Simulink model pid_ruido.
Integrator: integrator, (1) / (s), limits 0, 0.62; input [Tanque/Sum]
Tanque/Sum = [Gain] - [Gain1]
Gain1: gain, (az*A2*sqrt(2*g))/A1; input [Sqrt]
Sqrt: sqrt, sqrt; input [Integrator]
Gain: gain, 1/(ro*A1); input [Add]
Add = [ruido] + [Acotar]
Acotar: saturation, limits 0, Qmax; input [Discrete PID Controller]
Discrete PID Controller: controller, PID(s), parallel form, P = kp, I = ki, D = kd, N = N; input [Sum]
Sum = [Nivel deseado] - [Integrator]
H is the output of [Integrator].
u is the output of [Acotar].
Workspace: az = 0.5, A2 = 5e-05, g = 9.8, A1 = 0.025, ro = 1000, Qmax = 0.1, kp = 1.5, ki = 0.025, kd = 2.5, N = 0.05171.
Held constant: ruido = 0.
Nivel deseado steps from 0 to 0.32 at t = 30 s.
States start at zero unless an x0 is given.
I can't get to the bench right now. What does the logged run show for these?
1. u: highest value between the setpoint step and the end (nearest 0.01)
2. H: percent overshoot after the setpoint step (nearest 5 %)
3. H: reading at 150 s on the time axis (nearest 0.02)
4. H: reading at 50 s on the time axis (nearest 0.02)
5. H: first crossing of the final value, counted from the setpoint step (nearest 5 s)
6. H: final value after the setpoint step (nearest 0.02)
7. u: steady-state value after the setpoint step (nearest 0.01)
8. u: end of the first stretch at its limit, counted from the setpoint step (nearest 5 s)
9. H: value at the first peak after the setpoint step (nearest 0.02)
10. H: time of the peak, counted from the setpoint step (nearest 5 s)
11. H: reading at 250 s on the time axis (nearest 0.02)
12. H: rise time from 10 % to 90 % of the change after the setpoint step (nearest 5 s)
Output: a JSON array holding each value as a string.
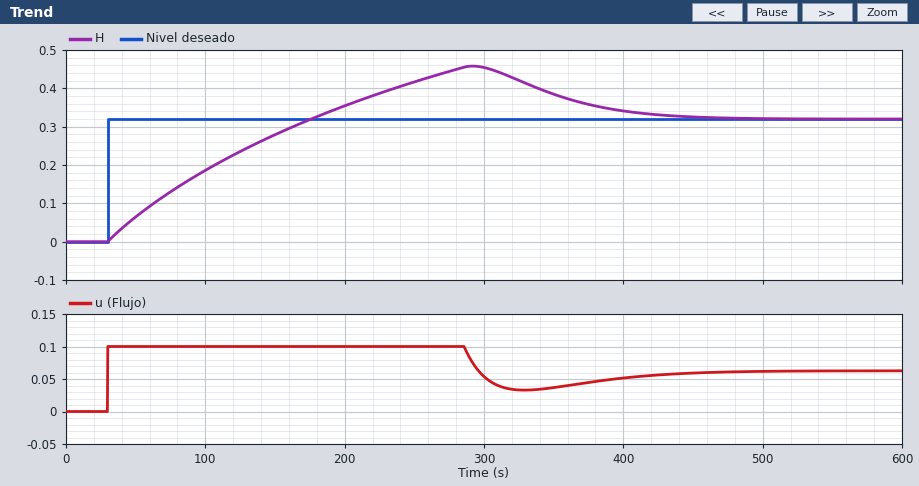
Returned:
["0.10", "45 %", "0.28", "0.06", "145 s", "0.32", "0.06", "255 s", "0.46", "260 s", "0.42", "115 s"]
